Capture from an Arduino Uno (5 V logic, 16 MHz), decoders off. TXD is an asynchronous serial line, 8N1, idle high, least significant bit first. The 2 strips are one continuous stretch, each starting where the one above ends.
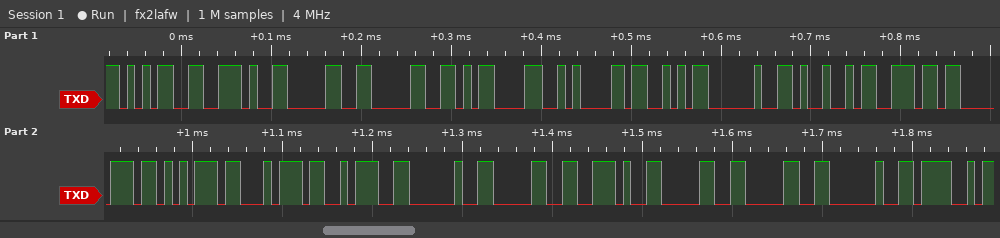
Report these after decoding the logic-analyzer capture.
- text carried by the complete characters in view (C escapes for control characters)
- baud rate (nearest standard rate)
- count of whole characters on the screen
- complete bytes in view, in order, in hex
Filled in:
"5.00\r\nS Input: 0.00 O"
115200 baud
21
0x35 0x2E 0x30 0x30 0x0D 0x0A 0x53 0x20 0x49 0x6E 0x70 0x75 0x74 0x3A 0x20 0x30 0x2E 0x30 0x30 0x20 0x4F
